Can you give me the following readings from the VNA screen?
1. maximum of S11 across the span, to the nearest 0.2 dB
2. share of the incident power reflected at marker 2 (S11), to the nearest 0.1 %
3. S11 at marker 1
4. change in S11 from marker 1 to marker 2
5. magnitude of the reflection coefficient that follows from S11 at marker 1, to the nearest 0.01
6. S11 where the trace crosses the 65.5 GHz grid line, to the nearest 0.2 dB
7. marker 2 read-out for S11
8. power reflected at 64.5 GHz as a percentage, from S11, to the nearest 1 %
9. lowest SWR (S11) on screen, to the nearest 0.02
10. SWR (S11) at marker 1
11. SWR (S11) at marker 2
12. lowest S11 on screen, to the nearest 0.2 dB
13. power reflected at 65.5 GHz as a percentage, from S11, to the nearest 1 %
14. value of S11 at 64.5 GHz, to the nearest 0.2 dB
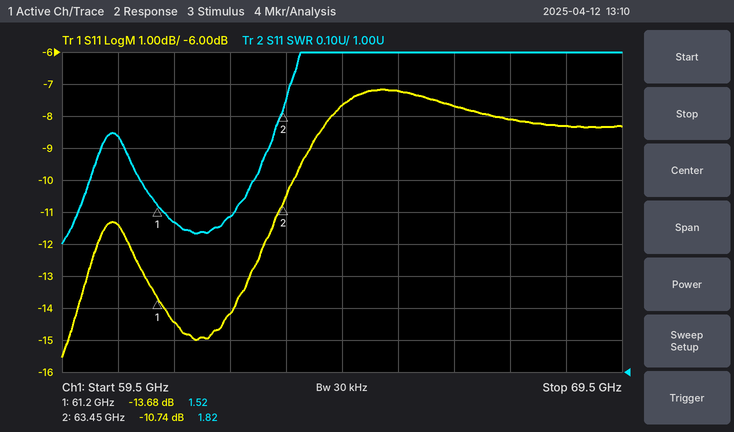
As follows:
-7.2 dB
8.4 %
-13.68 dB
2.94 dB
0.21
-7.2 dB
-10.74 dB
17 %
1.40
1.52
1.82
-15.6 dB
19 %
-7.6 dB
